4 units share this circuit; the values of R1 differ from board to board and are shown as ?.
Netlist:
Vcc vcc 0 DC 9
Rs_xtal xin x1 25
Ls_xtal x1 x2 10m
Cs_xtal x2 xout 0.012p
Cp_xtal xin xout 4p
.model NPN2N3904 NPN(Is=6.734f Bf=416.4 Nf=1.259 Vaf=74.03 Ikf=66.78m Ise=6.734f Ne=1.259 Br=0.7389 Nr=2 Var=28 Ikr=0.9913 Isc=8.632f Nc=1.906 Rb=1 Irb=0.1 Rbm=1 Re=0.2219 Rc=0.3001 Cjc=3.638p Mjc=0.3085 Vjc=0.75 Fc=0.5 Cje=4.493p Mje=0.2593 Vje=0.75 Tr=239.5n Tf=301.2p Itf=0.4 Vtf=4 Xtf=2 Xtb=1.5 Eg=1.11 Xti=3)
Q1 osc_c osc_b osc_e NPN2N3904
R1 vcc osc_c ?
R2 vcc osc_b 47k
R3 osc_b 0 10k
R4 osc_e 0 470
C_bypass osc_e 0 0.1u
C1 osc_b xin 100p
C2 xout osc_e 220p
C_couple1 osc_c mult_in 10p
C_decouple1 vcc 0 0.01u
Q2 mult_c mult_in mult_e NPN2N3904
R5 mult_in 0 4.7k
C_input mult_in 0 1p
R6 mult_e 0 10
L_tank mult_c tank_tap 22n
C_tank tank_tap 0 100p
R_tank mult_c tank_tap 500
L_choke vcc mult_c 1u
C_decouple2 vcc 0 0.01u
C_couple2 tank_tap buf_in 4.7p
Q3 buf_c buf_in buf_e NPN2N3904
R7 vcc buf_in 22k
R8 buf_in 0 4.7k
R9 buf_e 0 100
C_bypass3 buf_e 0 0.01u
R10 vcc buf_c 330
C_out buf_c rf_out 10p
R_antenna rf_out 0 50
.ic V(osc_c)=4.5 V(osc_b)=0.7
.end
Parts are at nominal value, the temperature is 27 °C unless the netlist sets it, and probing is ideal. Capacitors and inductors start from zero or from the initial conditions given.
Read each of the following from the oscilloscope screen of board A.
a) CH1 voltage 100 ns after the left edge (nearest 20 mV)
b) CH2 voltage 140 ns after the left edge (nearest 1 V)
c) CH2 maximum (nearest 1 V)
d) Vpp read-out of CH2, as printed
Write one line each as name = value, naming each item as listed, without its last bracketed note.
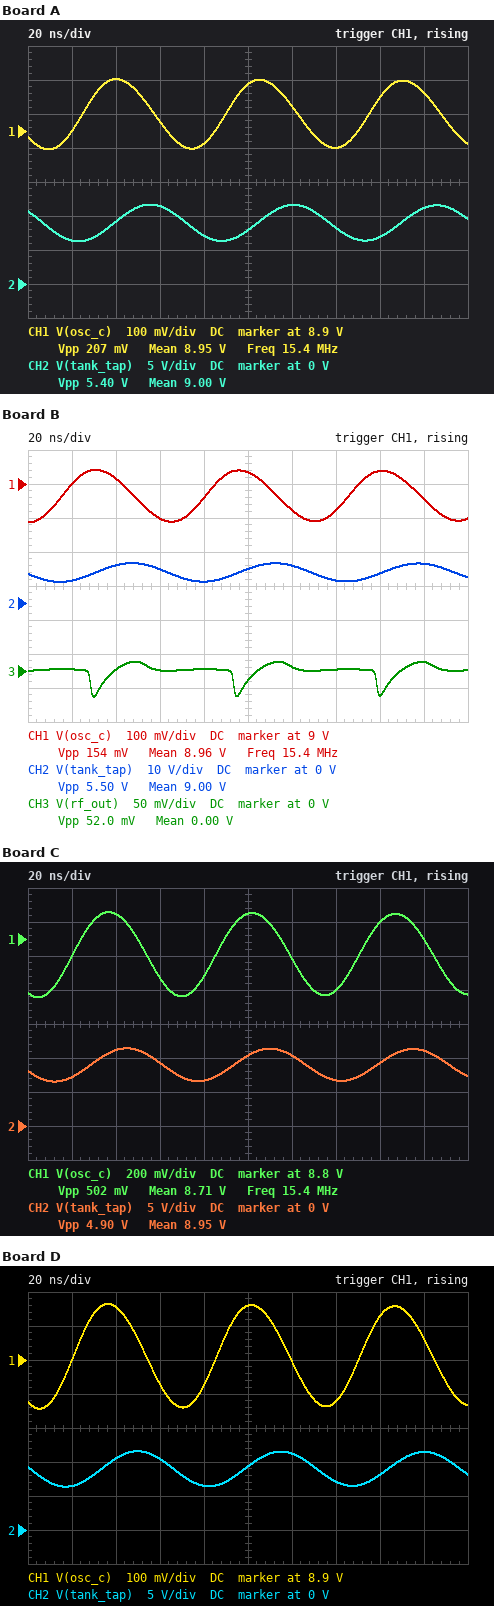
CH1 voltage 100 ns after the left edge = 9.04 V
CH2 voltage 140 ns after the left edge = 8 V
CH2 maximum = 12 V
Vpp read-out of CH2, as printed = 5.40 V
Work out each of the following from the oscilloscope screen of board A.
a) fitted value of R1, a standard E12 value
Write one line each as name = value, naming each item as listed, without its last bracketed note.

fitted value of R1, a standard E12 value = 470 Ω
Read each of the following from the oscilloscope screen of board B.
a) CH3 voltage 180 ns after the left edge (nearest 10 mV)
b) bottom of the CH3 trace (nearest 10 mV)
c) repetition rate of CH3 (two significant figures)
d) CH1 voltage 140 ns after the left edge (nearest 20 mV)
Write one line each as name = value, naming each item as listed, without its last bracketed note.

CH3 voltage 180 ns after the left edge = 10 mV
bottom of the CH3 trace = -40 mV
repetition rate of CH3 = 15 MHz
CH1 voltage 140 ns after the left edge = 8.92 V
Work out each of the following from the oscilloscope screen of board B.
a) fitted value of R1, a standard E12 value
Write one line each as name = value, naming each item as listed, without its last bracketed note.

fitted value of R1, a standard E12 value = 330 Ω
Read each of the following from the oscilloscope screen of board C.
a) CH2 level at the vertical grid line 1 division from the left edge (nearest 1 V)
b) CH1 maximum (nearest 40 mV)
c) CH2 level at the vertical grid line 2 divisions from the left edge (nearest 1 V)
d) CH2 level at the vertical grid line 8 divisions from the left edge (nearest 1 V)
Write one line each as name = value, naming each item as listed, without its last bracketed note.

CH2 level at the vertical grid line 1 division from the left edge = 7 V
CH1 maximum = 8.96 V
CH2 level at the vertical grid line 2 divisions from the left edge = 11 V
CH2 level at the vertical grid line 8 divisions from the left edge = 9 V
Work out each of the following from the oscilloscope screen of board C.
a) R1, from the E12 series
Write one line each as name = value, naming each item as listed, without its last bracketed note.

R1, from the E12 series = 2.7 kΩ
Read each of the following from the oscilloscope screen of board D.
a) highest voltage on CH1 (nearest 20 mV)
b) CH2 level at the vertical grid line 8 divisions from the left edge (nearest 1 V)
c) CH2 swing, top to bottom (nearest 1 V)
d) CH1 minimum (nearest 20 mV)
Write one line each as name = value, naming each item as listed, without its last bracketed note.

highest voltage on CH1 = 9.06 V
CH2 level at the vertical grid line 8 divisions from the left edge = 8 V
CH2 swing, top to bottom = 5 V
CH1 minimum = 8.76 V
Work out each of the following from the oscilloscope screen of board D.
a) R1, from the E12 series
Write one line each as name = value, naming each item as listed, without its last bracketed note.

R1, from the E12 series = 820 Ω
